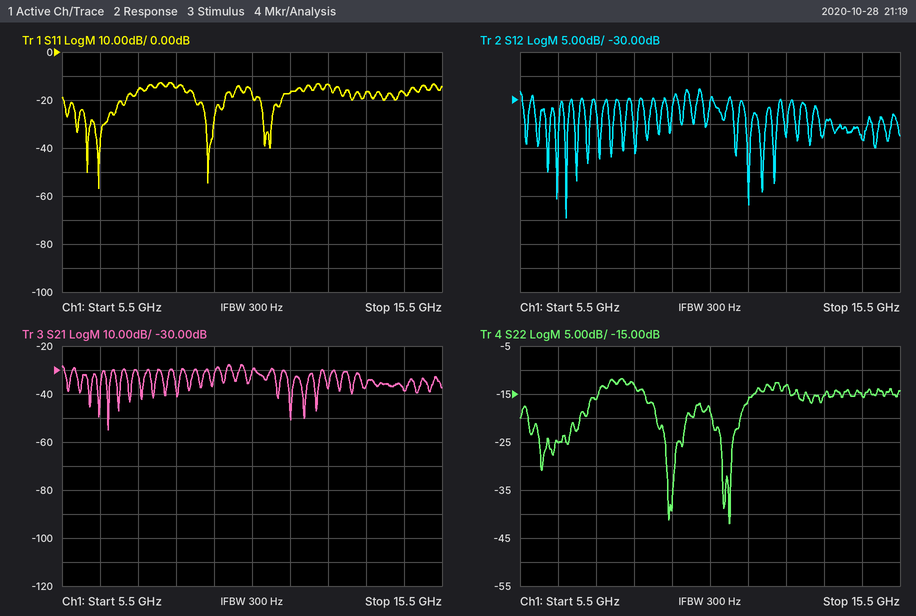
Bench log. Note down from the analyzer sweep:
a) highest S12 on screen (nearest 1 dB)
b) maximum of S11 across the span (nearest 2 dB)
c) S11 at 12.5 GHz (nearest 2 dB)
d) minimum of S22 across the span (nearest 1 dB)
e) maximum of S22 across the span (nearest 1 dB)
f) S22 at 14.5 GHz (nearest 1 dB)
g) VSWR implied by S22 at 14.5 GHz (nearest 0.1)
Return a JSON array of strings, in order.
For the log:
["-28 dB", "-12 dB", "-14 dB", "-42 dB", "-12 dB", "-15 dB", "1.4"]
